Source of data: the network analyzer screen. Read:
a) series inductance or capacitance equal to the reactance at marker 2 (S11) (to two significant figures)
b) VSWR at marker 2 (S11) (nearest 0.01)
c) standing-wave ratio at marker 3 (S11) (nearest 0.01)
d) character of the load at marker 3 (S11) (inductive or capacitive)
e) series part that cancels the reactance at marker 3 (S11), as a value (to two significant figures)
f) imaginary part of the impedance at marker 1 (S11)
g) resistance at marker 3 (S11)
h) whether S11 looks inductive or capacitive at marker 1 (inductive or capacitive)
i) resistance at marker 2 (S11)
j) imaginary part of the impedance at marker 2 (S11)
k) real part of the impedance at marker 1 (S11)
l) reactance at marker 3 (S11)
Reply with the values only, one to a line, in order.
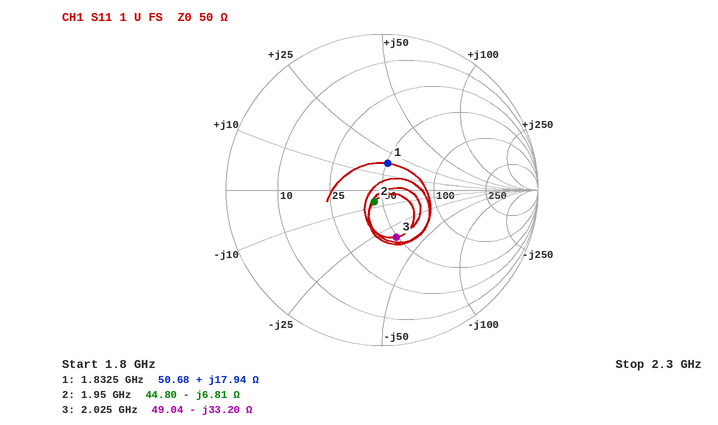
12 pF
1.20
1.93
capacitive
2.6 nH
+17.94 Ω
49.04 Ω
inductive
44.80 Ω
-6.81 Ω
50.68 Ω
-33.20 Ω
